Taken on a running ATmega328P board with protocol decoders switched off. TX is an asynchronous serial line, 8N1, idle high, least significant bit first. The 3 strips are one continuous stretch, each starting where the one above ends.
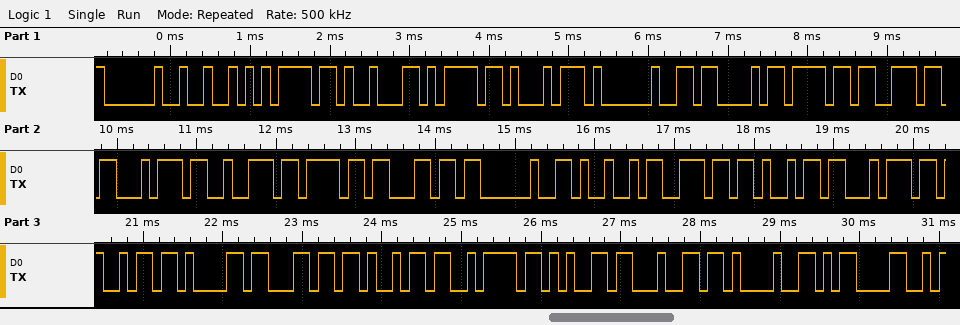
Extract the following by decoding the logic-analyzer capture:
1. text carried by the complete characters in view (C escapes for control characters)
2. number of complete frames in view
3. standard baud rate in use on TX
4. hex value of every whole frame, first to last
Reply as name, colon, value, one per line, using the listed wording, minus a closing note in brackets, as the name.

text carried by the complete characters in view: " Robot Control Initialized!\r"
number of complete frames in view: 28
standard baud rate in use on TX: 9600 baud
hex value of every whole frame, first to last: 0x20 0x52 0x6F 0x62 0x6F 0x74 0x20 0x43 0x6F 0x6E 0x74 0x72 0x6F 0x6C 0x20 0x49 0x6E 0x69 0x74 0x69 0x61 0x6C 0x69 0x7A 0x65 0x64 0x21 0x0D
